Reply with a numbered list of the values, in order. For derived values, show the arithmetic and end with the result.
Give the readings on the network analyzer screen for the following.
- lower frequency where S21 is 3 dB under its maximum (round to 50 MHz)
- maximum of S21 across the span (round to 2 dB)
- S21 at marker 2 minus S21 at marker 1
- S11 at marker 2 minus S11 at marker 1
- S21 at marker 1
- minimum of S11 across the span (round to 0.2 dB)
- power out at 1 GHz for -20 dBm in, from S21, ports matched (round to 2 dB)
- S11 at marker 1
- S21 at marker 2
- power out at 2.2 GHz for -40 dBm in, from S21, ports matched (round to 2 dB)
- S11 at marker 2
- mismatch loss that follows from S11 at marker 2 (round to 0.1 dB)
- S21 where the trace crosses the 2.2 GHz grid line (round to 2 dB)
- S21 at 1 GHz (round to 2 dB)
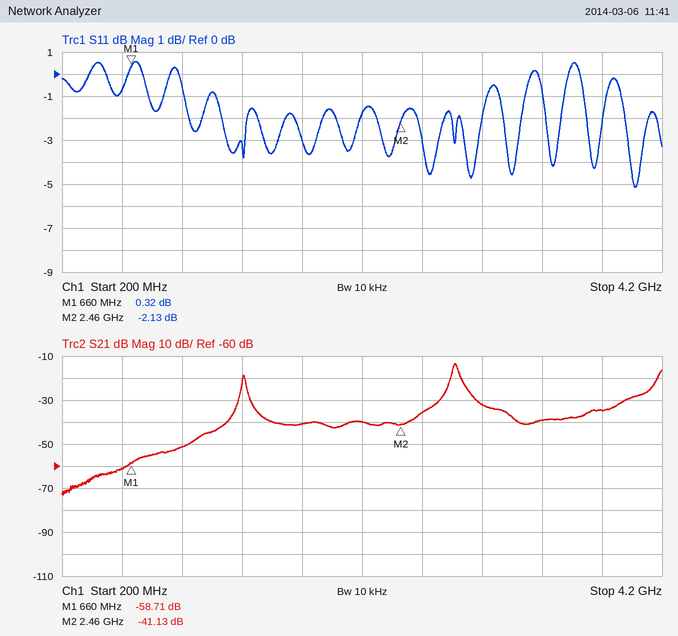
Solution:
1. 2.80 GHz
2. -14 dB
3. -41.13 − (-58.71) = 17.58 dB
4. -2.13 − (0.32) = -2.45 dB
5. -58.71 dB
6. -5.2 dB
7. -20 dBm + (-52 dB) = -72 dBm
8. 0.32 dB
9. -41.13 dB
10. -40 dBm + (-40 dB) = -80 dBm
11. -2.13 dB
12. −10 log10(1 − 10^(-2.13/10)) ≈ 4.1 dB
13. -40 dB
14. -52 dB
